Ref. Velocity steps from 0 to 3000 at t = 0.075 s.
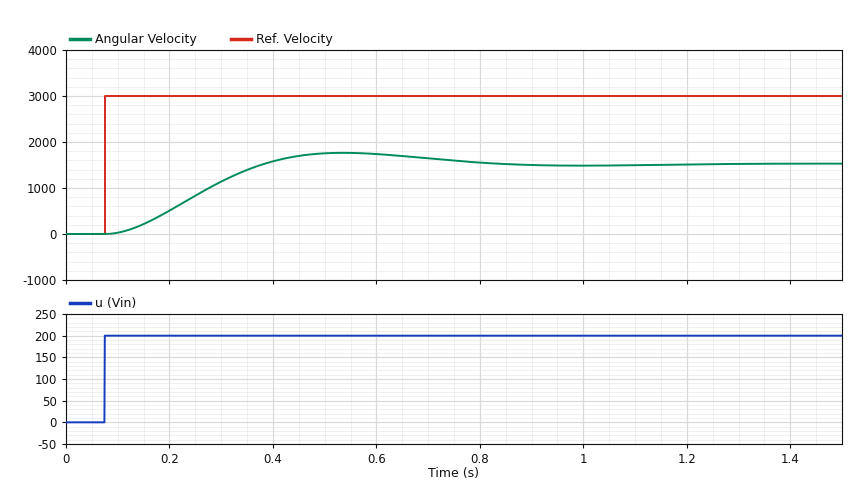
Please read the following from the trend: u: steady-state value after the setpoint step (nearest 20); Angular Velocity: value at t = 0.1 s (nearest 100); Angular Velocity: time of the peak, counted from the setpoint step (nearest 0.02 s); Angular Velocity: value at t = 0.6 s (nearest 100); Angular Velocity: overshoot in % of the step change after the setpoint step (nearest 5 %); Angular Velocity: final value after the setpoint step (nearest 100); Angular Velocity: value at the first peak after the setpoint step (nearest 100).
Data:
200
0
0.46 s
1700
15 %
1500
1800
